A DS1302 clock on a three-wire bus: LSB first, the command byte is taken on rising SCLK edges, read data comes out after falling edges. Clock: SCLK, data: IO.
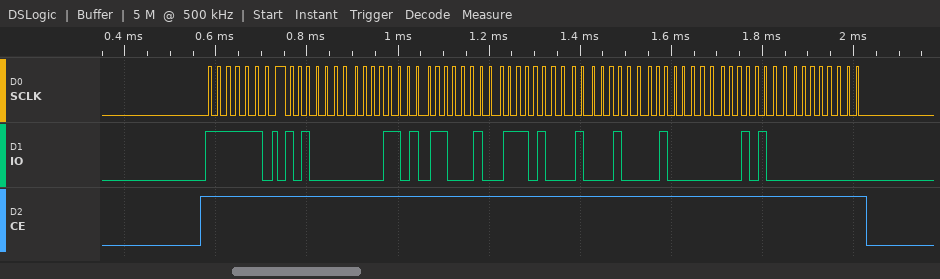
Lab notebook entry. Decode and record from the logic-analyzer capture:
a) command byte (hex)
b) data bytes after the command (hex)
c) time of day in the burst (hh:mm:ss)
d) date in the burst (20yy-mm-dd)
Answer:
0xBF
05 58 23 17 11 02 14 00
23:58:05
2014-11-17
